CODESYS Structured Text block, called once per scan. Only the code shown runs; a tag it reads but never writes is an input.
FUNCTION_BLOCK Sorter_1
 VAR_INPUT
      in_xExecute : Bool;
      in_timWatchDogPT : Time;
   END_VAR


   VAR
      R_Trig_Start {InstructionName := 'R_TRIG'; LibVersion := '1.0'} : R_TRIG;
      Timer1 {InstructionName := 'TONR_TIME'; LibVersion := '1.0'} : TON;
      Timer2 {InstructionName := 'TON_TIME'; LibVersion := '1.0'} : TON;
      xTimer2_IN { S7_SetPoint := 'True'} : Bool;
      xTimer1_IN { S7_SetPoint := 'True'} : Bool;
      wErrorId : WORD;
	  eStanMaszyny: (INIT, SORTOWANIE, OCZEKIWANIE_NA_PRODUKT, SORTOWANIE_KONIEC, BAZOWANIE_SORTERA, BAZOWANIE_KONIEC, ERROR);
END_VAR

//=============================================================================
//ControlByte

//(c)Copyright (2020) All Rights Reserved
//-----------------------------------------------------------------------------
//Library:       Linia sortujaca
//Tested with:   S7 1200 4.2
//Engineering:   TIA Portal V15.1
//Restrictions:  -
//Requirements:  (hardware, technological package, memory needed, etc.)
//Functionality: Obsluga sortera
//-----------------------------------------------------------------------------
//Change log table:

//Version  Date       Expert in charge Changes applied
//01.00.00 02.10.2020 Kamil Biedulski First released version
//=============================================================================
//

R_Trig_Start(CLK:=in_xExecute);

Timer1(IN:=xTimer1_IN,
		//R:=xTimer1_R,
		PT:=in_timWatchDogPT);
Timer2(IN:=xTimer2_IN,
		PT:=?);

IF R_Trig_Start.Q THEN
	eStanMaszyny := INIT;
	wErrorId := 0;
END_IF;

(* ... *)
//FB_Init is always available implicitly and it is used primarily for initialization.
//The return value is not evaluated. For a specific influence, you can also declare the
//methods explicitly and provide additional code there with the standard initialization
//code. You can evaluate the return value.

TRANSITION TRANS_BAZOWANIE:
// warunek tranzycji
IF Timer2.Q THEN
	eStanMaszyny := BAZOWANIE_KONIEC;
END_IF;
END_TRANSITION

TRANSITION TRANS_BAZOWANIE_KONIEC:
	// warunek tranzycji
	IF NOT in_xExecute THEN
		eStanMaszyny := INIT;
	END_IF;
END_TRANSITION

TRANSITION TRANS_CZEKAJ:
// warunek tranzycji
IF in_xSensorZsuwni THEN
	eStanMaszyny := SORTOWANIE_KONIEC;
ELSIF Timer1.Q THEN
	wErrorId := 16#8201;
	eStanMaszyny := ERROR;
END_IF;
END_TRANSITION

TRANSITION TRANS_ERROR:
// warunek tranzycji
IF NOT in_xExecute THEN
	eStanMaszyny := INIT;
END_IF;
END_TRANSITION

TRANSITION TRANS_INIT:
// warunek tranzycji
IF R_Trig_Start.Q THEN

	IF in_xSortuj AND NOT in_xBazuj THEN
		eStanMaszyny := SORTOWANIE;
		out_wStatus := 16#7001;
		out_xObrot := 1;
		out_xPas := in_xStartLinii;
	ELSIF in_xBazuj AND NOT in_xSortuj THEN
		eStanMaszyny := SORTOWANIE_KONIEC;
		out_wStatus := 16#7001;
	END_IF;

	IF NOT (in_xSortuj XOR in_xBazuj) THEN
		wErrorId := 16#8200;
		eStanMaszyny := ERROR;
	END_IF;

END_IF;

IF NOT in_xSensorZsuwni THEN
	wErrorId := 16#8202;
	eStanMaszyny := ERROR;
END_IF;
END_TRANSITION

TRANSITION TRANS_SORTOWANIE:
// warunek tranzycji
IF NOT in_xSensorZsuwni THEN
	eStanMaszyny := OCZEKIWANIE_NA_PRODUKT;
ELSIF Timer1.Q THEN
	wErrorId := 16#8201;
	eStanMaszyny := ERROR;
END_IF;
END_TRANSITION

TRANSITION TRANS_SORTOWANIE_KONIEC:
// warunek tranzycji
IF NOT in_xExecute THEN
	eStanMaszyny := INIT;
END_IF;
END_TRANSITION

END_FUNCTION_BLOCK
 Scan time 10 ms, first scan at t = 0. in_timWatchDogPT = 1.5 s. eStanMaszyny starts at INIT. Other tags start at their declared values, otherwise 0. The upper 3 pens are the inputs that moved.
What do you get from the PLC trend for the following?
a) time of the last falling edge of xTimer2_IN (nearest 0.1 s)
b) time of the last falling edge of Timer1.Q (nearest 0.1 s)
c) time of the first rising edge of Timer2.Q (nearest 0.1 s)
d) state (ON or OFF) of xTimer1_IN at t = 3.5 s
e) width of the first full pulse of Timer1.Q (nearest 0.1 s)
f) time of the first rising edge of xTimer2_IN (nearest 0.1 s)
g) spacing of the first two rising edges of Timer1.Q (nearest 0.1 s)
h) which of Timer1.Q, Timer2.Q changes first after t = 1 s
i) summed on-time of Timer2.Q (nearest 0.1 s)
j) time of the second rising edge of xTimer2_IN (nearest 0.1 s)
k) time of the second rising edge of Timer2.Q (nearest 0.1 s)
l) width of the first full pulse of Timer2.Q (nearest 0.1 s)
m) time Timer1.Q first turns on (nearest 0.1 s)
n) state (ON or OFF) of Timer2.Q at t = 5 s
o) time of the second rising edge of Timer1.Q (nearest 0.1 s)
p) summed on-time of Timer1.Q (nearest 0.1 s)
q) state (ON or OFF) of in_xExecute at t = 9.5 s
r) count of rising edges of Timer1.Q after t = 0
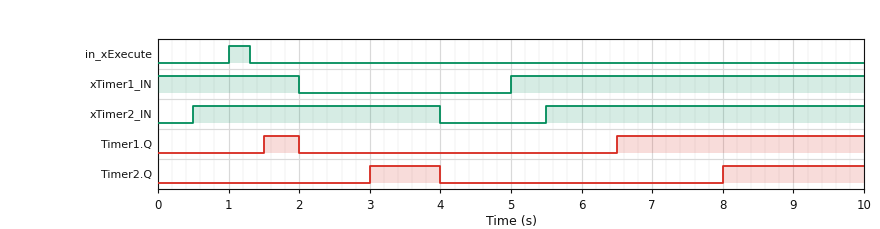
4.0 s
2.0 s
3.0 s
OFF
0.5 s
0.5 s
5.0 s
Timer1.Q
3.0 s
5.5 s
8.0 s
1.0 s
1.5 s
OFF
6.5 s
4.0 s
OFF
2
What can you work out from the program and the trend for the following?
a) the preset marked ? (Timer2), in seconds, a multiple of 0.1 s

2.5 s
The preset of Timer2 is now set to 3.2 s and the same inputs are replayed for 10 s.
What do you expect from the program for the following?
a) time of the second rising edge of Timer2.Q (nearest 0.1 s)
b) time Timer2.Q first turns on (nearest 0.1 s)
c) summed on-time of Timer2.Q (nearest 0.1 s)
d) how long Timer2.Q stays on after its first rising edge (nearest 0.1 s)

8.7 s
3.7 s
1.6 s
0.3 s
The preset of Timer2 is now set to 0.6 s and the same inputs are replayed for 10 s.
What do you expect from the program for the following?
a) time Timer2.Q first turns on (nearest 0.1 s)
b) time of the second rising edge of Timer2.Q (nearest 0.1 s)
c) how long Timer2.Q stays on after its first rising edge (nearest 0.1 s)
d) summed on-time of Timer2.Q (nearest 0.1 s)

1.1 s
6.1 s
2.9 s
6.8 s
